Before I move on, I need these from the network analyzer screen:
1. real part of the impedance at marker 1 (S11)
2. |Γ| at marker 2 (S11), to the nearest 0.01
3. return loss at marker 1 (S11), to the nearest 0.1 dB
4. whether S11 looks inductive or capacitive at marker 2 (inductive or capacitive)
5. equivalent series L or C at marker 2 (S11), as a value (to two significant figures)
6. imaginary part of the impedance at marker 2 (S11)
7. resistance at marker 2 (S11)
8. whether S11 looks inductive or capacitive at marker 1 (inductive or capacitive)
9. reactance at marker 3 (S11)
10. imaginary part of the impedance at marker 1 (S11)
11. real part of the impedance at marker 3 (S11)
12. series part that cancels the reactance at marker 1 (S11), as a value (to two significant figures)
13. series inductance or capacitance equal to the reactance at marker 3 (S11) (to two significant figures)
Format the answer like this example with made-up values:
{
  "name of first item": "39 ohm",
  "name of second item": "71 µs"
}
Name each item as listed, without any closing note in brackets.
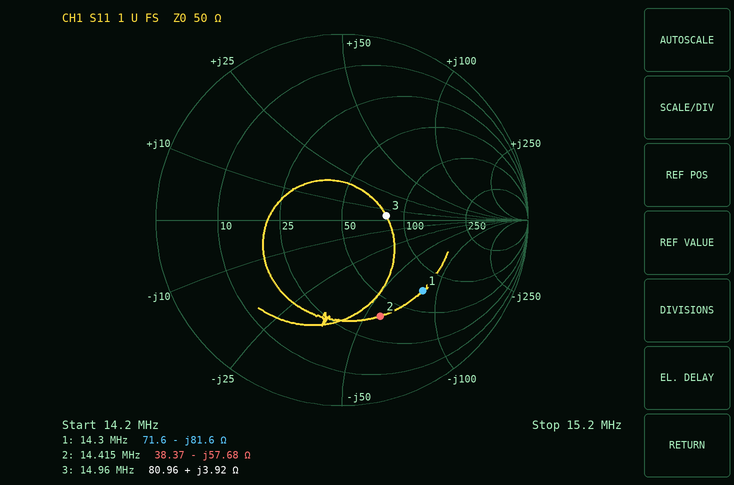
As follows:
{
  "real part of the impedance at marker 1": "71.6 Ω",
  "|Γ| at marker 2 (S11), to the nearest 0.01": "0.56",
  "return loss at marker 1 (S11), to the nearest 0.1 dB": "4.8 dB",
  "whether S11 looks inductive or capacitive at marker 2": "capacitive",
  "equivalent series L or C at marker 2 (S11), as a value": "190 pF",
  "imaginary part of the impedance at marker 2": "-57.68 Ω",
  "resistance at marker 2": "38.37 Ω",
  "whether S11 looks inductive or capacitive at marker 1": "capacitive",
  "reactance at marker 3": "+3.92 Ω",
  "imaginary part of the impedance at marker 1": "-81.6 Ω",
  "real part of the impedance at marker 3": "80.96 Ω",
  "series part that cancels the reactance at marker 1 (S11), as a value": "910 nH",
  "series inductance or capacitance equal to the reactance at marker 3 (S11)": "42 nH"
}
